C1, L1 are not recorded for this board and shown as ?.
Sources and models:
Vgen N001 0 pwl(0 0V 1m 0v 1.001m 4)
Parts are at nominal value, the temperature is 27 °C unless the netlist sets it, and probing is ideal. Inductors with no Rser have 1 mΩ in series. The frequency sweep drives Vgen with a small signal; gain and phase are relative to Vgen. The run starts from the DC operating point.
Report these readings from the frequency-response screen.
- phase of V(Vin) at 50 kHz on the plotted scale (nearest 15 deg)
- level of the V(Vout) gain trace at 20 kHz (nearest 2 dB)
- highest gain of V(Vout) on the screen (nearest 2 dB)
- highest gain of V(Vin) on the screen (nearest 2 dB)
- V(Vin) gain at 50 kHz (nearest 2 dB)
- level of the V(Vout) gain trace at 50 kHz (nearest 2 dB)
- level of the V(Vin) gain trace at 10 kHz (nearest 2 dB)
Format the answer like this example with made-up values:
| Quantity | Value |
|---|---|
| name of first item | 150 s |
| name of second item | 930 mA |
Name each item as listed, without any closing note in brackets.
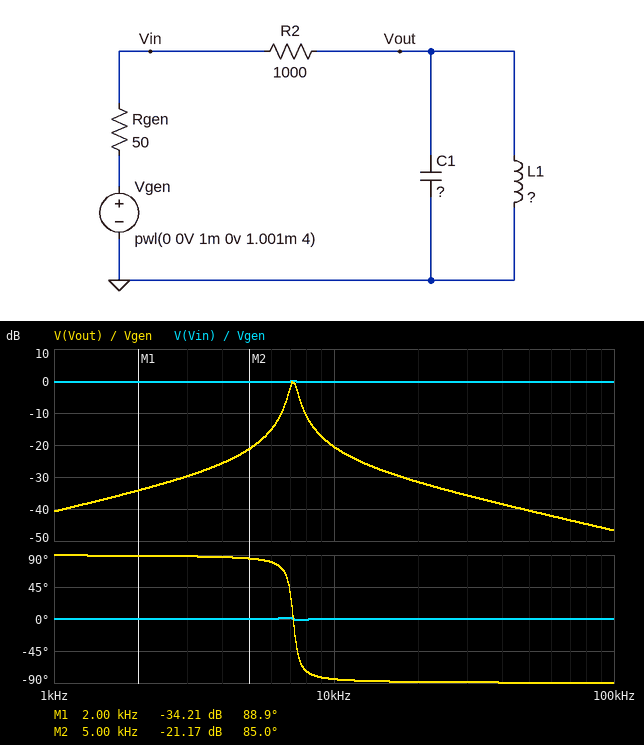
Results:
| Quantity | Value |
|---|---|
| phase of V(Vin) at 50 kHz on the plotted scale | 0 deg |
| level of the V(Vout) gain trace at 20 kHz | -32 dB |
| highest gain of V(Vout) on the screen | 0 dB |
| highest gain of V(Vin) on the screen | 0 dB |
| V(Vin) gain at 50 kHz | 0 dB |
| level of the V(Vout) gain trace at 50 kHz | -40 dB |
| level of the V(Vin) gain trace at 10 kHz | 0 dB |
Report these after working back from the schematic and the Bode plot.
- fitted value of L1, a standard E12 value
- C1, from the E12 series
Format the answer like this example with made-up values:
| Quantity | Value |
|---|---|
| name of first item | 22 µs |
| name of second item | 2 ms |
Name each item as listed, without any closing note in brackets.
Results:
| Quantity | Value |
|---|---|
| fitted value of L1, a standard E12 value | 1.5 mH |
| C1, from the E12 series | 330 nF |
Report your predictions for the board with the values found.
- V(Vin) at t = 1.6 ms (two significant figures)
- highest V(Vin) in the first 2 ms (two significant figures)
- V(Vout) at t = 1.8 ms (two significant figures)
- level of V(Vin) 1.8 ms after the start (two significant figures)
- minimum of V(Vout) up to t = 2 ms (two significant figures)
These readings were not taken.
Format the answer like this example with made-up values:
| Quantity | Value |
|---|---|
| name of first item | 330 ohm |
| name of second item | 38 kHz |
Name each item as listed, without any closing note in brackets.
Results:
| Quantity | Value |
|---|---|
| V(Vin) at t = 1.6 ms | 3.8 V |
| highest V(Vin) in the first 2 ms | 3.8 V |
| V(Vout) at t = 1.8 ms | -79 mV |
| level of V(Vin) 1.8 ms after the start | 3.8 V |
| minimum of V(Vout) up to t = 2 ms | -220 mV |
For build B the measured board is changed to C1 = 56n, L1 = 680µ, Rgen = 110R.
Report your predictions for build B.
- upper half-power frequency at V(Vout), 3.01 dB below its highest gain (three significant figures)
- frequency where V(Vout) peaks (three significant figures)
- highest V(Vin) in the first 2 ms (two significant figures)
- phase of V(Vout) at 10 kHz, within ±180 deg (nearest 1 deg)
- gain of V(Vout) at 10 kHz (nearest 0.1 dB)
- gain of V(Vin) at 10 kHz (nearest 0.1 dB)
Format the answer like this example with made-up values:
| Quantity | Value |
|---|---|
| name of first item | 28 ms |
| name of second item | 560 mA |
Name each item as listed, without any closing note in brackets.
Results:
| Quantity | Value |
|---|---|
| upper half-power frequency at V(Vout), 3.01 dB below its highest gain | 27.1 kHz |
| frequency where V(Vout) peaks | 25.8 kHz |
| highest V(Vin) in the first 2 ms | 3.6 V |
| phase of V(Vout) at 10 kHz, within ±180 deg | 87 deg |
| gain of V(Vout) at 10 kHz | -26.9 dB |
| gain of V(Vin) at 10 kHz | -0.9 dB |
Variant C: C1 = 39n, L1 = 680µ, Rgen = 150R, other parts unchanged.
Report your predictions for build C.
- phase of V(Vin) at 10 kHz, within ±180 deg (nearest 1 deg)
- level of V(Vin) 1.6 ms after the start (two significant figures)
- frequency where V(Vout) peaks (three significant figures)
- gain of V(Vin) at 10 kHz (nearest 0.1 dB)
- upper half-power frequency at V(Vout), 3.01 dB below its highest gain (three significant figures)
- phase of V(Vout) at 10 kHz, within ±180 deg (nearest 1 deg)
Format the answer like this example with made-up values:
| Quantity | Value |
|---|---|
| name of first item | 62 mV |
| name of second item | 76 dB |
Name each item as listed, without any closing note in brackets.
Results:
| Quantity | Value |
|---|---|
| phase of V(Vin) at 10 kHz, within ±180 deg | 0 deg |
| level of V(Vin) 1.6 ms after the start | 3.5 V |
| frequency where V(Vout) peaks | 30.9 kHz |
| gain of V(Vin) at 10 kHz | -1.2 dB |
| upper half-power frequency at V(Vout), 3.01 dB below its highest gain | 32.7 kHz |
| phase of V(Vout) at 10 kHz, within ±180 deg | 88 deg |
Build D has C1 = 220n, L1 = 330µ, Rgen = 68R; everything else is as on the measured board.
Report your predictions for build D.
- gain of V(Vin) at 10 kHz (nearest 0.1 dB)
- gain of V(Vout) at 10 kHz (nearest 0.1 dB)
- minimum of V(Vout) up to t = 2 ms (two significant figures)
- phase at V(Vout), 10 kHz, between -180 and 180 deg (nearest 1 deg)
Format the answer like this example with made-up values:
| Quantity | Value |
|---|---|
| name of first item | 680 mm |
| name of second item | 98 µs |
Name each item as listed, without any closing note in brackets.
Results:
| Quantity | Value |
|---|---|
| gain of V(Vin) at 10 kHz | -0.6 dB |
| gain of V(Vout) at 10 kHz | -31.3 dB |
| minimum of V(Vout) up to t = 2 ms | -130 mV |
| phase at V(Vout), 10 kHz, between -180 and 180 deg | 88 deg |
